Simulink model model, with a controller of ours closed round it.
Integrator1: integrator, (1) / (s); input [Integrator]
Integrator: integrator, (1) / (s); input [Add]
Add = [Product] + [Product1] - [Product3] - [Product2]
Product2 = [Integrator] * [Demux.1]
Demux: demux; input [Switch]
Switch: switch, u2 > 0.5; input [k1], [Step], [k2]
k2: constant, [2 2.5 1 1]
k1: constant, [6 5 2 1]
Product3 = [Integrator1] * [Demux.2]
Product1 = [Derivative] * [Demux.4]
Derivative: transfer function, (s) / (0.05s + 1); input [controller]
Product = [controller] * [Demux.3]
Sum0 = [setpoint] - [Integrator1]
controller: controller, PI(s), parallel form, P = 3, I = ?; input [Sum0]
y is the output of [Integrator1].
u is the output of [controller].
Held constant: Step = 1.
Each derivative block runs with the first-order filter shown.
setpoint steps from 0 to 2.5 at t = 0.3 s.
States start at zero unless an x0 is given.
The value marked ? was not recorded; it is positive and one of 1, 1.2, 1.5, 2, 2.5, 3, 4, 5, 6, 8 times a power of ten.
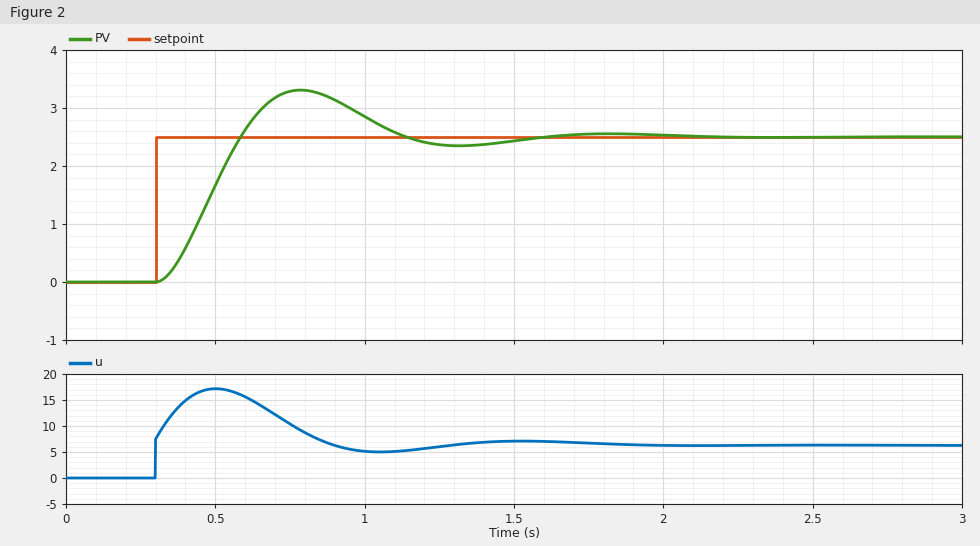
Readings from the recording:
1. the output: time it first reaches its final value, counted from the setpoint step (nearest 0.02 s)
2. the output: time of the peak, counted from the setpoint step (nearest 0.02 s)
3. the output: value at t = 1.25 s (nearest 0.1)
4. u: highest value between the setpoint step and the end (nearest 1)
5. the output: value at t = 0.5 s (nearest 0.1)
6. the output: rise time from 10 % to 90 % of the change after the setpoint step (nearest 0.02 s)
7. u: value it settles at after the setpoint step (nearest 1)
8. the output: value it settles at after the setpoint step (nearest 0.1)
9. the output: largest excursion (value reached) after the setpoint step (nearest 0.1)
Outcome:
0.28 s
0.48 s
2.4
17
1.7
0.20 s
6
2.5
3.3
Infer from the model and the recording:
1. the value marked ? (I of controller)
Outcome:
40
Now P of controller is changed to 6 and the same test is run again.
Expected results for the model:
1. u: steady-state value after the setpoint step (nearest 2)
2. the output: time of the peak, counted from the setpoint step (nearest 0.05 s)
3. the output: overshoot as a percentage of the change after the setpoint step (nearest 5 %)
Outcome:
6
0.40 s
15 %
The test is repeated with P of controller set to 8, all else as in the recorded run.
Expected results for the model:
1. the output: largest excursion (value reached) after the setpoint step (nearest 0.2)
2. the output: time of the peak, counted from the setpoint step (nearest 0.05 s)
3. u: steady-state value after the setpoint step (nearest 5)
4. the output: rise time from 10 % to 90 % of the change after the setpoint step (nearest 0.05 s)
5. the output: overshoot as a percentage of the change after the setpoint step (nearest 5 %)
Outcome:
2.8
0.35 s
5
0.15 s
10 %
